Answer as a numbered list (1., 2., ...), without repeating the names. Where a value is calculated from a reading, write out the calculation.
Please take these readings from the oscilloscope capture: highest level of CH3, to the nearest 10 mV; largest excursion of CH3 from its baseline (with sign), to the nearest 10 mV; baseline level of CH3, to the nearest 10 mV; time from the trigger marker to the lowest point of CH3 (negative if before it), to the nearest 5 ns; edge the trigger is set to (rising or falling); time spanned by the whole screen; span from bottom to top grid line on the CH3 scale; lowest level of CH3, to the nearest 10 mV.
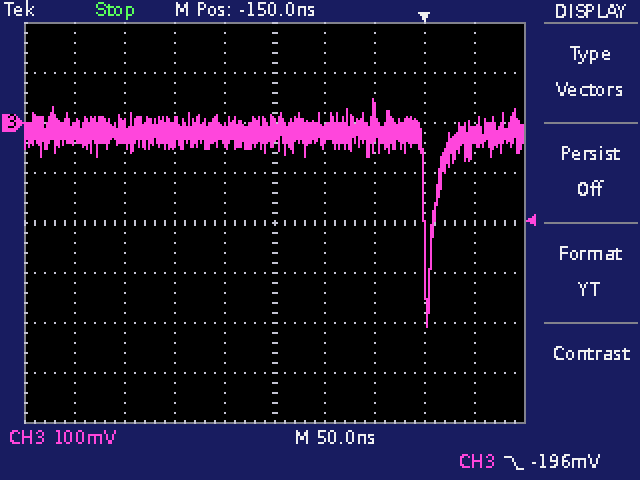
1. 50 mV
2. -410 mV − (-20 mV) = -390 mV
3. -20 mV
4. +5 ns
5. falling
6. 500 ns
7. 800 mV
8. -410 mV
